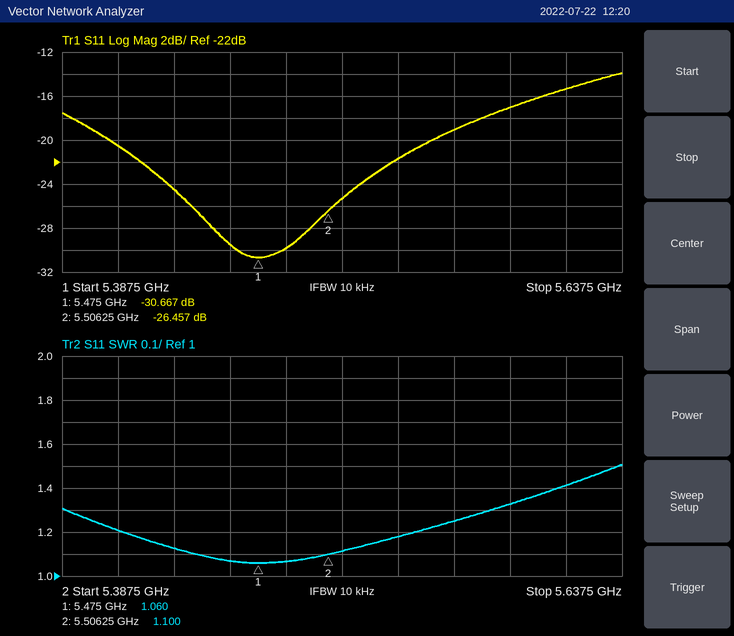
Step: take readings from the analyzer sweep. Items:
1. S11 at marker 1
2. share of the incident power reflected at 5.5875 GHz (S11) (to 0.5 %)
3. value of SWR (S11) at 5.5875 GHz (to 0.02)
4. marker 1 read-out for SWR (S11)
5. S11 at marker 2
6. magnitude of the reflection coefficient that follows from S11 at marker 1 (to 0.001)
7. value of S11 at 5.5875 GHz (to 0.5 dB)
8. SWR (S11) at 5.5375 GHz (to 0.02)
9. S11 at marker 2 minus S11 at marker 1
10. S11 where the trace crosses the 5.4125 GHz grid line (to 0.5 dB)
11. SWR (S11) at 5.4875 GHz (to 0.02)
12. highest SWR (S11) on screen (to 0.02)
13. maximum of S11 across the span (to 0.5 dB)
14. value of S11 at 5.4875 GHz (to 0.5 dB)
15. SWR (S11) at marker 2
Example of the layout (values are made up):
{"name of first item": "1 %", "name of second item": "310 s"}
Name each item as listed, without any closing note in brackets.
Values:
{"S11 at marker 1": "-30.667 dB", "share of the incident power reflected at 5.5875 GHz (S11)": "2.0 %", "value of SWR (S11) at 5.5875 GHz": "1.32", "marker 1 read-out for SWR": "1.060", "S11 at marker 2": "-26.457 dB", "magnitude of the reflection coefficient that follows from S11 at marker 1": "0.029", "value of S11 at 5.5875 GHz": "-17.0 dB", "SWR (S11) at 5.5375 GHz": "1.18", "S11 at marker 2 minus S11 at marker 1": "4.210 dB", "S11 where the trace crosses the 5.4125 GHz grid line": "-20.5 dB", "SWR (S11) at 5.4875 GHz": "1.06", "highest SWR (S11) on screen": "1.50", "maximum of S11 across the span": "-14.0 dB", "value of S11 at 5.4875 GHz": "-30.0 dB", "SWR (S11) at marker 2": "1.100"}
